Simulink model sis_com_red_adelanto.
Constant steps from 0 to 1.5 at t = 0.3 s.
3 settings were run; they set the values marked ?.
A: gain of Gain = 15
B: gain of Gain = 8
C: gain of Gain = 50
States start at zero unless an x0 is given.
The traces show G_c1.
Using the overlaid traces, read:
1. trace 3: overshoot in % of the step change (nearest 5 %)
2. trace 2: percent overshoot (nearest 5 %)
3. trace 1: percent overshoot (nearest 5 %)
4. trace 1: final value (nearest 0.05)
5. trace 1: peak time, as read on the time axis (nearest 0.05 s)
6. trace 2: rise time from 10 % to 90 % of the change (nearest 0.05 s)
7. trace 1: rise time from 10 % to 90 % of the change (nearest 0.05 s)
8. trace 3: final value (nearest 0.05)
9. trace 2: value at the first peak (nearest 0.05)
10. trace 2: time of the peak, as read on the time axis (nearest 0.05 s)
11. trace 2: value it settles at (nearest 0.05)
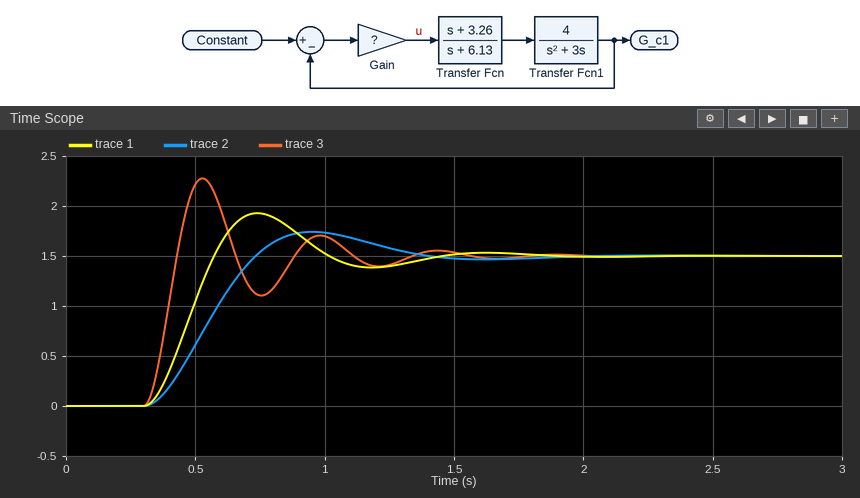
50 %
15 %
30 %
1.50
0.75 s
0.30 s
0.20 s
1.50
1.75
0.95 s
1.50
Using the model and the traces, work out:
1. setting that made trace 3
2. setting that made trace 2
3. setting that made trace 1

C
B
A
